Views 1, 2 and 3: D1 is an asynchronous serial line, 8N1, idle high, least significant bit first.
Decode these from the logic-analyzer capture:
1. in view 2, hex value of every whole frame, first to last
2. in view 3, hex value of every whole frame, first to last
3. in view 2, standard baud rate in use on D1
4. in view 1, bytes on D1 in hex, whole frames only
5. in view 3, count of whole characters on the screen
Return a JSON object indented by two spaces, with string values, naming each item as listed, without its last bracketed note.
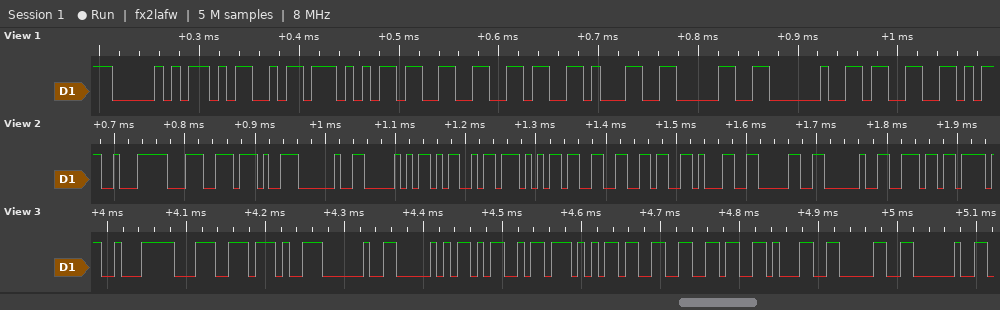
{
  "in view 2, hex value of every whole frame, first to last": "E2 9C 97 20 50 4D 57 33 36 31 30 20 6E",
  "in view 3, hex value of every whole frame, first to last": "0xE2 0x9C 0x97 0x20 0x50 0x4D 0x57 0x33 0x36 0x31 0x30 0x20",
  "in view 2, standard baud rate in use on D1": "115200 baud",
  "in view 1, bytes on D1 in hex, whole frames only": "0x50 0x4D 0x57 0x33 0x36 0x31 0x30 0x20 0x33",
  "in view 3, count of whole characters on the screen": "12"
}
